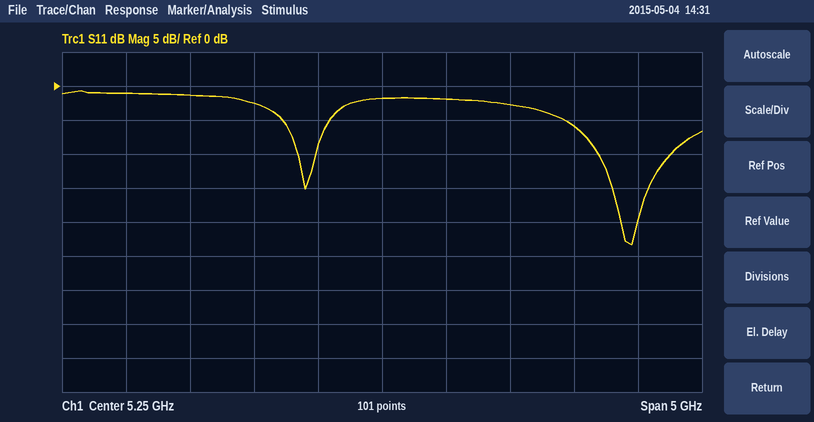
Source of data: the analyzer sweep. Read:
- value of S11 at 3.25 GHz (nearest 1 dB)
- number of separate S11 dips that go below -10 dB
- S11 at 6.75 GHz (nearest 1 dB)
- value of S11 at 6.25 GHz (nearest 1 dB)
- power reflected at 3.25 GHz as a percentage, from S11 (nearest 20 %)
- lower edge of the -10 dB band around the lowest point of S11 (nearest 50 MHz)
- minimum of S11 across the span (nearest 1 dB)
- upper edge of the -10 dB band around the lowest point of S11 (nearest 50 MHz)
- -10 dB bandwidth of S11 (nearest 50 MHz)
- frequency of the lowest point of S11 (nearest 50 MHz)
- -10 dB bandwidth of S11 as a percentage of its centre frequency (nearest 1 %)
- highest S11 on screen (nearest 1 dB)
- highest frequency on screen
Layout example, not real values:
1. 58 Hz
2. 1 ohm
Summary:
1. -1 dB
2. 2
3. -6 dB
4. -3 dB
5. 80 %
6. 6.95 GHz
7. -23 dB
8. 7.50 GHz
9. 550 MHz
10. 7.20 GHz
11. 8 %
12. -1 dB
13. 7.75 GHz
